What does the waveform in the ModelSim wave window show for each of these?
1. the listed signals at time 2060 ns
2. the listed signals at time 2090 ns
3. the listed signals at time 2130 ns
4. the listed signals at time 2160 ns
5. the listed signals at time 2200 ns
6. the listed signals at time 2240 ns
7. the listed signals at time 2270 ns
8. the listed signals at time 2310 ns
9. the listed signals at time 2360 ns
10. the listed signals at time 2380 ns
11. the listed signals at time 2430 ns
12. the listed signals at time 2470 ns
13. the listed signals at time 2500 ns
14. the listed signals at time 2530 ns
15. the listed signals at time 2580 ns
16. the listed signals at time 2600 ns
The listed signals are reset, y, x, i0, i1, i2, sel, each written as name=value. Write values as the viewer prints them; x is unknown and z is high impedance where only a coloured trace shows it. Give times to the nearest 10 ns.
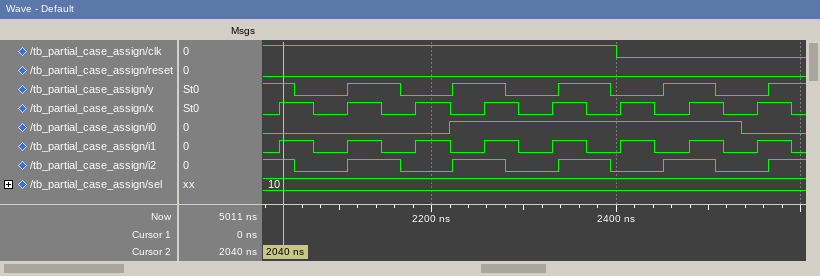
reset=0, y=0, x=1, i0=0, i1=1, i2=0, sel=10
reset=0, y=0, x=0, i0=0, i1=0, i2=0, sel=10
reset=0, y=1, x=1, i0=0, i1=1, i2=1, sel=10
reset=0, y=1, x=0, i0=0, i1=0, i2=1, sel=10
reset=0, y=0, x=1, i0=0, i1=1, i2=0, sel=10
reset=0, y=1, x=0, i0=1, i1=0, i2=1, sel=10
reset=0, y=1, x=1, i0=1, i1=1, i2=1, sel=10
reset=0, y=0, x=0, i0=1, i1=0, i2=0, sel=10
reset=0, y=1, x=1, i0=1, i1=1, i2=1, sel=10
reset=0, y=1, x=0, i0=1, i1=0, i2=1, sel=10
reset=0, y=0, x=1, i0=1, i1=1, i2=0, sel=10
reset=0, y=1, x=0, i0=1, i1=0, i2=1, sel=10
reset=0, y=1, x=1, i0=1, i1=1, i2=1, sel=10
reset=0, y=0, x=0, i0=1, i1=0, i2=0, sel=10
reset=0, y=1, x=1, i0=0, i1=1, i2=1, sel=10
reset=0, y=1, x=0, i0=0, i1=0, i2=1, sel=10
